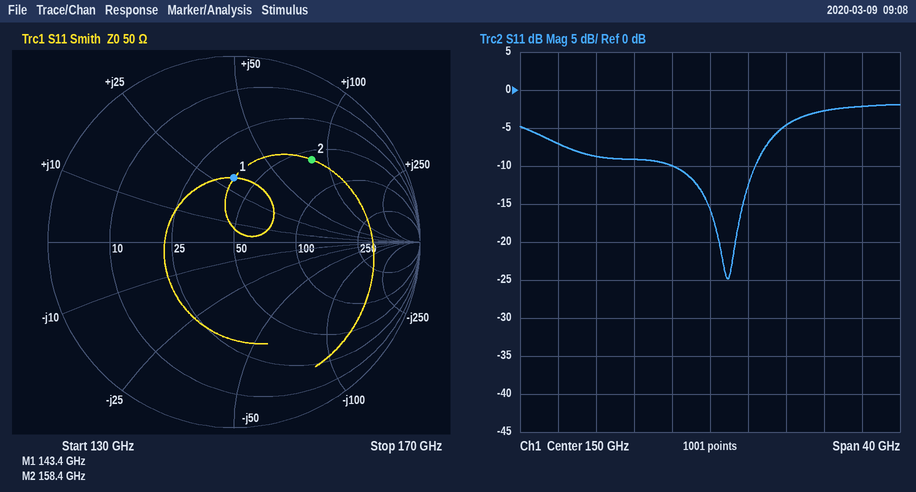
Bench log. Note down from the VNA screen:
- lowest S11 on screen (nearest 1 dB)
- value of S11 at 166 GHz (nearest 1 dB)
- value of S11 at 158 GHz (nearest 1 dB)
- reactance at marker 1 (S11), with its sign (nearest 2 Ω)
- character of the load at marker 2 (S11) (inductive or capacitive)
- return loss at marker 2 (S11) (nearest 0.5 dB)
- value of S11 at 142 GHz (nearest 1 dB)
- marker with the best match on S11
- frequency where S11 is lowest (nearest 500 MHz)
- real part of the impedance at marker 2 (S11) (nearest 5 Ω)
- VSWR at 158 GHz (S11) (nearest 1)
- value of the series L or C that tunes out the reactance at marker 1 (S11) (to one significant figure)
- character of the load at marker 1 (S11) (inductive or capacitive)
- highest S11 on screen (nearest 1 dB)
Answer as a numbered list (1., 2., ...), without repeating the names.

1. -25 dB
2. -2 dB
3. -5 dB
4. +30 Ω
5. inductive
6. 4.5 dB
7. -9 dB
8. marker 1
9. 152.0 GHz
10. 60 Ω
11. 4
12. 40 fF
13. inductive
14. -2 dB
